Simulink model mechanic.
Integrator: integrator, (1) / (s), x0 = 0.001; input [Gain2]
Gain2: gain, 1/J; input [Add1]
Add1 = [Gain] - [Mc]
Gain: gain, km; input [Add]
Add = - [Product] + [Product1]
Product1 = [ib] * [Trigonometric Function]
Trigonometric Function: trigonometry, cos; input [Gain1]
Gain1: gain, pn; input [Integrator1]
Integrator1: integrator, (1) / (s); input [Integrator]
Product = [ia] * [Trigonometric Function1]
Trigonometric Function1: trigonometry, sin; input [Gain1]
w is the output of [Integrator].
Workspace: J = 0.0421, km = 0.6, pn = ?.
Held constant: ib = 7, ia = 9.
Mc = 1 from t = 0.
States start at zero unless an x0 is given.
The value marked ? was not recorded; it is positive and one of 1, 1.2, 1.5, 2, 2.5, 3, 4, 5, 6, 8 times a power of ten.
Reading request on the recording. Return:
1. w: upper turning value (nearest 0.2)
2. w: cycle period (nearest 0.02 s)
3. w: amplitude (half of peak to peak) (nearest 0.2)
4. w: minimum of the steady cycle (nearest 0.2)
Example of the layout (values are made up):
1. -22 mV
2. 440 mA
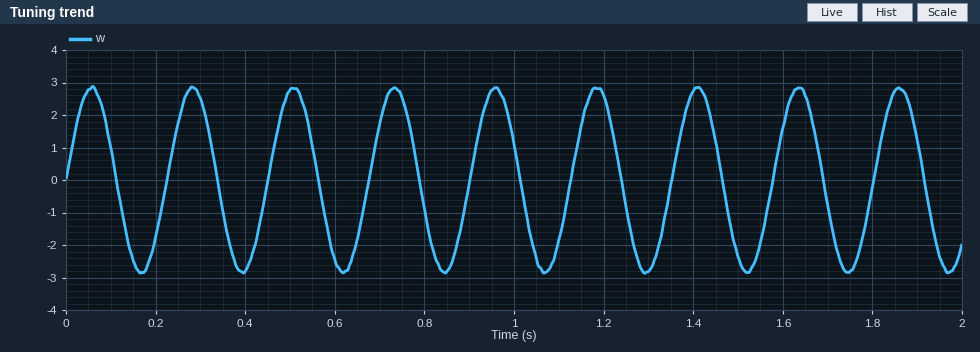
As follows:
1. 2.8
2. 0.22 s
3. 2.8
4. -2.8
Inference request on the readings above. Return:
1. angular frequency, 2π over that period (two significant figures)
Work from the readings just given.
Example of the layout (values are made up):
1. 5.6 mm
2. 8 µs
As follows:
1. 29 rad/s
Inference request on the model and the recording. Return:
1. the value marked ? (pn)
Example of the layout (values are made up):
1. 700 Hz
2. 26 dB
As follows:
1. 5
